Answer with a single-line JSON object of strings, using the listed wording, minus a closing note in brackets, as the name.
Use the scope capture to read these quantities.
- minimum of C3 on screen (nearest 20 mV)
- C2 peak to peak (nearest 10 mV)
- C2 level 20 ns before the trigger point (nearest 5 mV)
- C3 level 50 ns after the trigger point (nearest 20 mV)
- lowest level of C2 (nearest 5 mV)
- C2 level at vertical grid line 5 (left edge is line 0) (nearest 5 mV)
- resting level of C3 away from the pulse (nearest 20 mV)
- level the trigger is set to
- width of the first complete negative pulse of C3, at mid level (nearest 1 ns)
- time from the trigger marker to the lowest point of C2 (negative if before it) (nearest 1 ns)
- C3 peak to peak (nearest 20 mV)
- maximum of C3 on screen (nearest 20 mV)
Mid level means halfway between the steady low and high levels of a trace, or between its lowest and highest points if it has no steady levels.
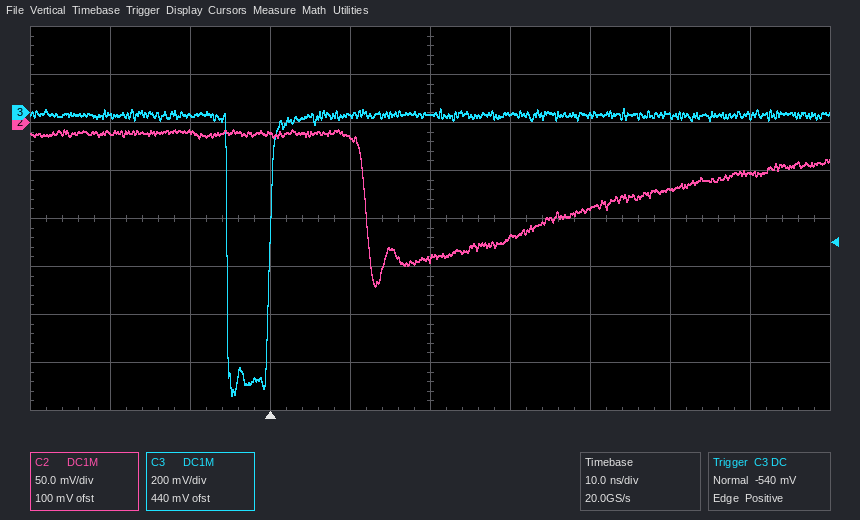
{"minimum of C3 on screen": "-1.18 V", "C2 peak to peak": "160 mV", "C2 level 20 ns before the trigger point": "-10 mV", "C3 level 50 ns after the trigger point": "-20 mV", "lowest level of C2": "-170 mV", "C2 level at vertical grid line 5 (left edge is line 0)": "-140 mV", "resting level of C3 away from the pulse": "0 mV", "level the trigger is set to": "-540 mV", "width of the first complete negative pulse of C3, at mid level": "5 ns", "time from the trigger marker to the lowest point of C2 (negative if before it)": "+13 ns", "C3 peak to peak": "1.20 V", "maximum of C3 on screen": "20 mV"}
